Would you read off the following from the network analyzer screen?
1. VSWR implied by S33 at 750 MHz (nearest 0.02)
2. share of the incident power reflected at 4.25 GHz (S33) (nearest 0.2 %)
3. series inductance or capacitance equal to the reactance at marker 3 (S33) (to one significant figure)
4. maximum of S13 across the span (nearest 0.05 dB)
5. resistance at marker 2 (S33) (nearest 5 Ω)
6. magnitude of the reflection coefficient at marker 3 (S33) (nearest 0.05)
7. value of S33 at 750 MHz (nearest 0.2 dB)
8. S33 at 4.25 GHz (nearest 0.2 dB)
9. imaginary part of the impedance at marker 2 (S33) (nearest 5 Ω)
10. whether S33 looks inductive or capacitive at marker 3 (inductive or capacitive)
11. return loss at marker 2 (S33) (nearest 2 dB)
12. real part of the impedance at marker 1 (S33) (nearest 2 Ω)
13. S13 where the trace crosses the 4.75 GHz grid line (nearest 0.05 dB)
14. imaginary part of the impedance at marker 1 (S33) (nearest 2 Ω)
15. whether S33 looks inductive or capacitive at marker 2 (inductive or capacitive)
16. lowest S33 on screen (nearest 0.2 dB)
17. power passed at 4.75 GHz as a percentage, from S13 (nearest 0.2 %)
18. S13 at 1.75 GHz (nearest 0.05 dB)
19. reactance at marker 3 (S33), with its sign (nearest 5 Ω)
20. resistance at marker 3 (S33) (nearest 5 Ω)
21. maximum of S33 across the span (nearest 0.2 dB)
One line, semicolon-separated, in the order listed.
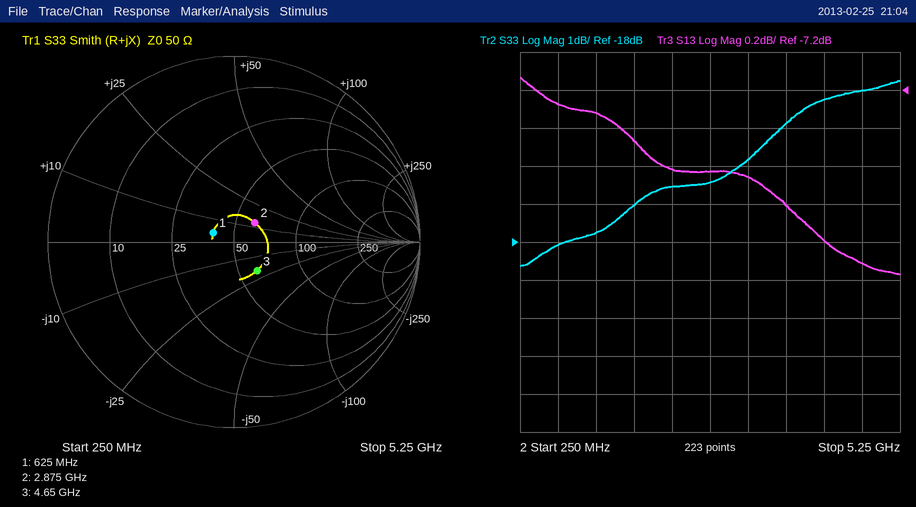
1.28; 3.8 %; 2 pF; -7.15 dB; 60 Ω; 0.20; -18.0 dB; -14.2 dB; +15 Ω; capacitive; 16 dB; 40 Ω; -8.10 dB; +4 Ω; inductive; -18.6 dB; 15.4 %; -7.45 dB; -20 Ω; 60 Ω; -13.8 dB
